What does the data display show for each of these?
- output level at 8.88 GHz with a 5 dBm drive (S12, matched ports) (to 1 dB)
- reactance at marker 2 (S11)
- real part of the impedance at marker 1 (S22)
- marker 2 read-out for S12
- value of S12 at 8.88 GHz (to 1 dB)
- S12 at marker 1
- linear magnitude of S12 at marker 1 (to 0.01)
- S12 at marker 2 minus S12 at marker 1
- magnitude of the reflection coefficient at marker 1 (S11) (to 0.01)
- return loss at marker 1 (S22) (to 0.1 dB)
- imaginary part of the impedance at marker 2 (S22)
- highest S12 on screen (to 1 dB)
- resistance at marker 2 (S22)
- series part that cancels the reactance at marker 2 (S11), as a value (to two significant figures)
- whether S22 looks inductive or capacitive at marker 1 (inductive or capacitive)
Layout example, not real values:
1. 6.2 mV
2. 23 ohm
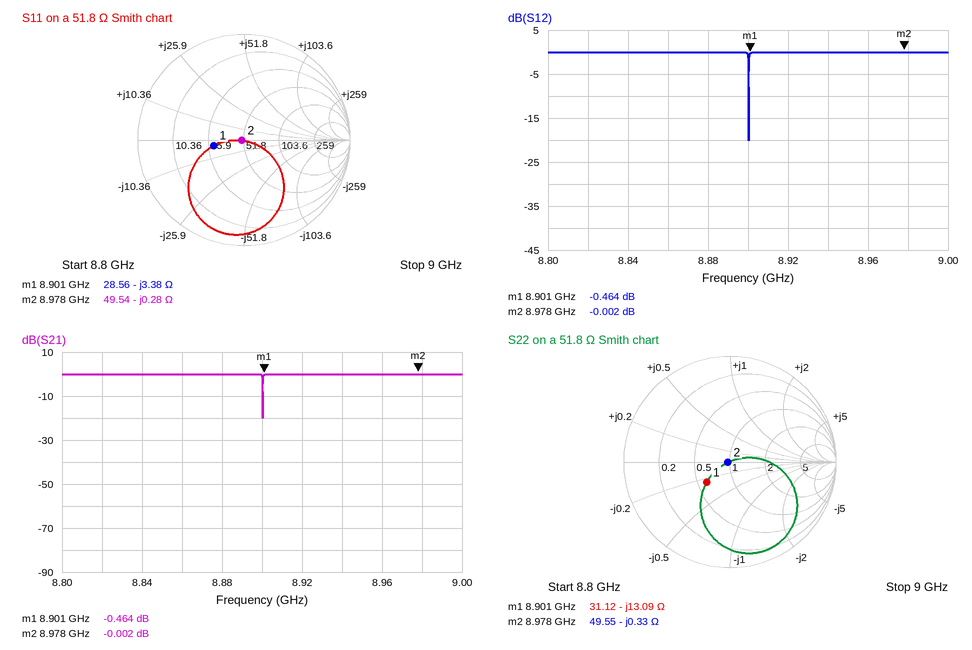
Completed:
1. 5 dBm
2. -0.28 Ω
3. 31.12 Ω
4. -0.002 dB
5. 0 dB
6. -0.464 dB
7. 0.95
8. 0.462 dB
9. 0.29
10. 10.7 dB
11. -0.33 Ω
12. 0 dB
13. 49.55 Ω
14. 5.0 pH
15. capacitive
